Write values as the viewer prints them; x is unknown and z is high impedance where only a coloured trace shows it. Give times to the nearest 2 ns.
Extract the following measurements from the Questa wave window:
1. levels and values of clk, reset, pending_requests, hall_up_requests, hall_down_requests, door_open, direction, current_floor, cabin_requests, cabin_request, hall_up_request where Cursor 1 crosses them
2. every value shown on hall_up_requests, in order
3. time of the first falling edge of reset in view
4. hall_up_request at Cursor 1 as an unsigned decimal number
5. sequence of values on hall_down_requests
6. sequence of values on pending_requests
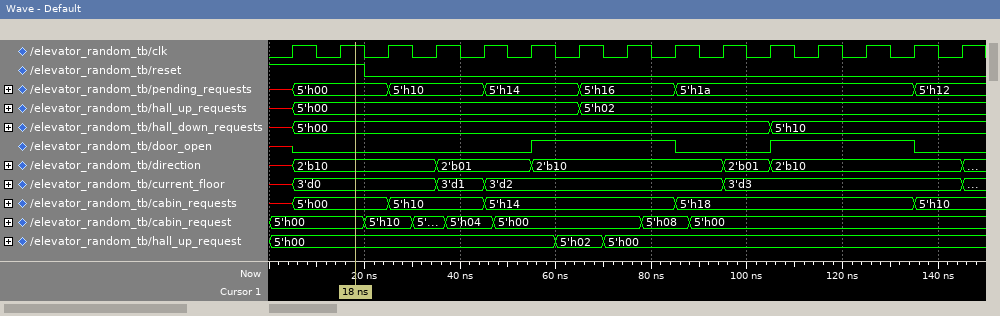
clk=1, reset=1, pending_requests=5'h00, hall_up_requests=5'h00, hall_down_requests=5'h00, door_open=0, direction=2'b10, current_floor=3'd0, cabin_requests=5'h00, cabin_request=5'h00, hall_up_request=5'h00
x, 5'h00, 5'h02
20 ns
0
x, 5'h00, 5'h10
x, 5'h00, 5'h10, 5'h14, 5'h16, 5'h1a, 5'h12
